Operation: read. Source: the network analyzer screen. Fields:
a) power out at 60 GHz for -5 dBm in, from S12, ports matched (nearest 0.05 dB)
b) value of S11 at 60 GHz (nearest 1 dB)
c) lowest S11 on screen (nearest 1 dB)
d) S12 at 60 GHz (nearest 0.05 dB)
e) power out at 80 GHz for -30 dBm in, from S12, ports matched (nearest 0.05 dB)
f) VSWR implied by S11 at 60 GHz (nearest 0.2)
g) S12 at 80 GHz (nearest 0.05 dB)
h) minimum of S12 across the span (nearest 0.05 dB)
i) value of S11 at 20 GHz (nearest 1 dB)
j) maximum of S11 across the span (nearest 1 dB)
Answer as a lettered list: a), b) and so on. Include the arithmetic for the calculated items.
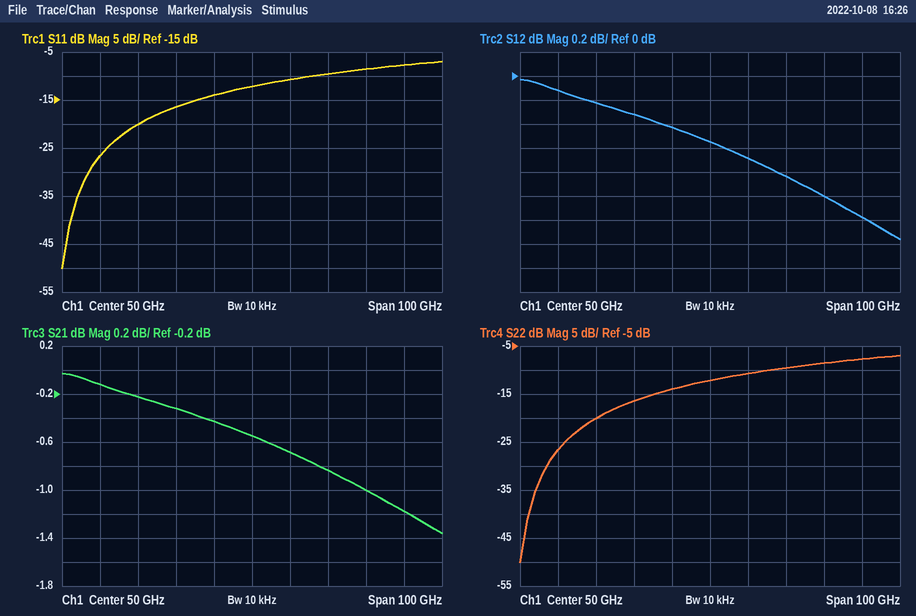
a) -5 dBm + (-0.70 dB) = -5.70 dBm
b) -11 dB
c) -50 dB
d) -0.70 dB
e) -30 dBm + (-1.00 dB) = -31.00 dBm
f) |Γ| = 10^(-11/20) = 0.2818; VSWR = (1 + 0.2818)/(1 − 0.2818) ≈ 1.8
g) -1.00 dB
h) -1.35 dB
i) -20 dB
j) -7 dB
